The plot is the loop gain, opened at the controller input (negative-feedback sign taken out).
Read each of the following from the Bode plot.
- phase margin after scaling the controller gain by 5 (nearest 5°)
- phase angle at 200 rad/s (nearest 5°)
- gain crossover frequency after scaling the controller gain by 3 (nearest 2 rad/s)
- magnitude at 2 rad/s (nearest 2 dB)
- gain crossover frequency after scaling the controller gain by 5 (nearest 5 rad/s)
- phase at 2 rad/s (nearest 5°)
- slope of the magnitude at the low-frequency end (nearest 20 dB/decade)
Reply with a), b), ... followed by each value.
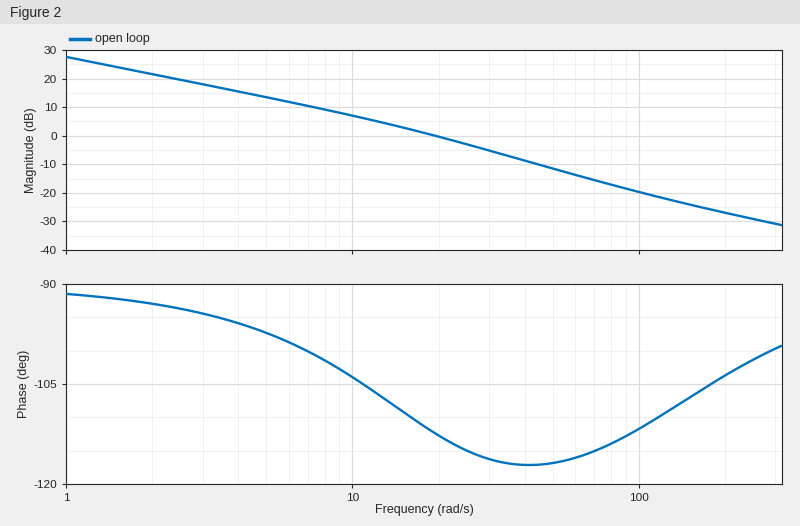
a) 65°
b) -105°
c) 42 rad/s
d) 22 dB
e) 60 rad/s
f) -95°
g) -20 dB/decade
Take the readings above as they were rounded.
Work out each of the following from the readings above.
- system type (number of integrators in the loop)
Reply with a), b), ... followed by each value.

a) 1
